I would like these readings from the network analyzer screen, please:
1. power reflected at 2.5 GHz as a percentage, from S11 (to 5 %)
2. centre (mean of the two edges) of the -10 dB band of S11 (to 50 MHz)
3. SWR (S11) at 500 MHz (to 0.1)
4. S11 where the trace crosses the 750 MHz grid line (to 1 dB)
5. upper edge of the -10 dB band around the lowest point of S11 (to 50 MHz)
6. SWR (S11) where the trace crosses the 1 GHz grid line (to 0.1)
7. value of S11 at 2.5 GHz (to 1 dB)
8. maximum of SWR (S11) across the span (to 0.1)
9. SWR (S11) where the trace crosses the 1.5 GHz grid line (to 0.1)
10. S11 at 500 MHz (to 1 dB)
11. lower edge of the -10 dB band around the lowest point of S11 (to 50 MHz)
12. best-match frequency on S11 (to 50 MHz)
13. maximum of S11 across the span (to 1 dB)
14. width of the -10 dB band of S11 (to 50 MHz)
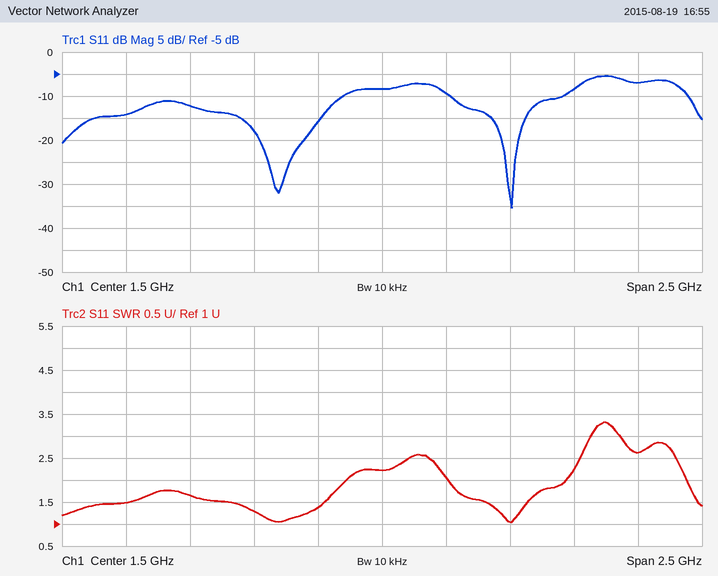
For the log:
20 %
2.00 GHz
1.5
-12 dB
2.20 GHz
1.3
-7 dB
3.3
2.2
-14 dB
1.75 GHz
2.00 GHz
-5 dB
450 MHz
